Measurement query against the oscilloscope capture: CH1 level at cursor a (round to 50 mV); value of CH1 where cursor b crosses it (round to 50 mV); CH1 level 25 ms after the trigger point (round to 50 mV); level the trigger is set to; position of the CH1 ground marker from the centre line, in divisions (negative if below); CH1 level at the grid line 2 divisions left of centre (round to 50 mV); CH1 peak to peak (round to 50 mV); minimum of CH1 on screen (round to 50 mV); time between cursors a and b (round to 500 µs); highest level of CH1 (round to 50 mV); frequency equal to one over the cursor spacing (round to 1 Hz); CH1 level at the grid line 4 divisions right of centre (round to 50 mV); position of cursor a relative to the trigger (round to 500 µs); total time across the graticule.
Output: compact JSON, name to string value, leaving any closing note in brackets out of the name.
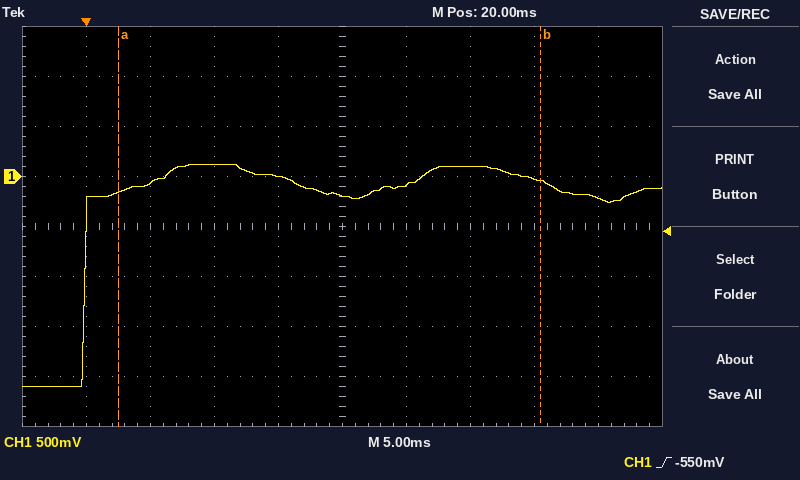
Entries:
{"CH1 level at cursor a": "-150 mV", "value of CH1 where cursor b crosses it": "-50 mV", "CH1 level 25 ms after the trigger point": "-100 mV", "level the trigger is set to": "-550 mV", "position of the CH1 ground marker from the centre line, in divisions": "+1.0 div", "CH1 level at the grid line 2 divisions left of centre": "100 mV", "CH1 peak to peak": "2.20 V", "minimum of CH1 on screen": "-2.10 V", "time between cursors a and b": "33.0 ms", "highest level of CH1": "100 mV", "frequency equal to one over the cursor spacing": "30 Hz", "CH1 level at the grid line 4 divisions right of centre": "-200 mV", "position of cursor a relative to the trigger": "+2.5 ms", "total time across the graticule": "50 ms"}
